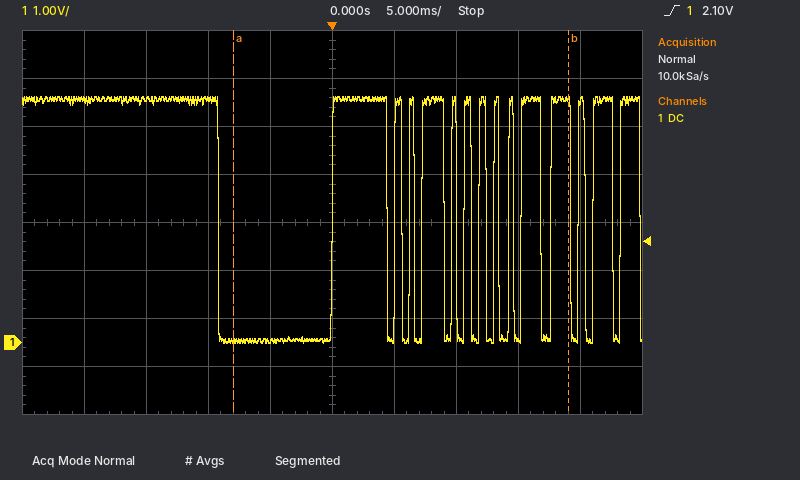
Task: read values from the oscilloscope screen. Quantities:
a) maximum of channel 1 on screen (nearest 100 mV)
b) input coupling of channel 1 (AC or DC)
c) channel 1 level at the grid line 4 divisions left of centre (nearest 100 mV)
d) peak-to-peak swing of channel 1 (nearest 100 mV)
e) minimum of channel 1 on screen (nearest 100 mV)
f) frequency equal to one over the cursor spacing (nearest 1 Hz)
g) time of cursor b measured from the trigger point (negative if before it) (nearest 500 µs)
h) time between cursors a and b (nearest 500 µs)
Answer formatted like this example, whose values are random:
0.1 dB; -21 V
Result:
5.1 V; DC; 5.1 V; 5.1 V; 0.0 V; 37 Hz; +19.0 ms; 27.0 ms
